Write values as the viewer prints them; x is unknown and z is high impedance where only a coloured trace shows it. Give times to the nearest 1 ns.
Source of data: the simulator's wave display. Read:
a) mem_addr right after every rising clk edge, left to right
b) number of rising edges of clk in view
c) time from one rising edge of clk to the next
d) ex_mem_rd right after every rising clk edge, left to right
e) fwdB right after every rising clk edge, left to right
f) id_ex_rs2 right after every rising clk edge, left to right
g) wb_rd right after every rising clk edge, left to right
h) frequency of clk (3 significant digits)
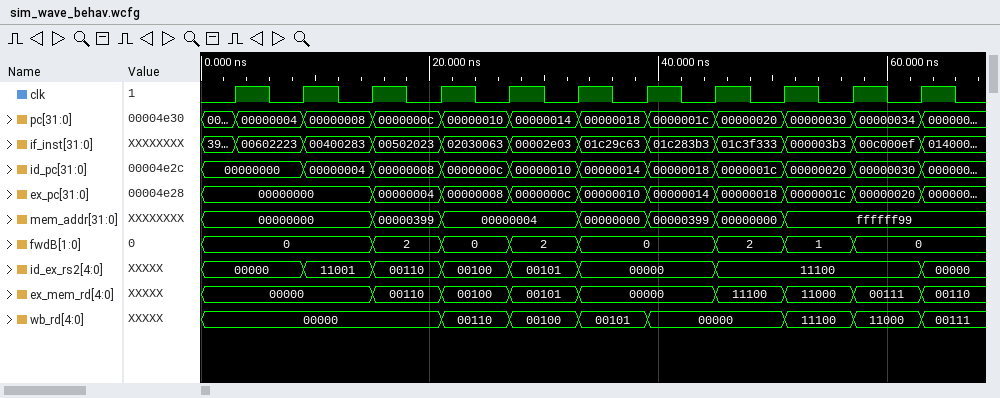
00000000, 00000000, 00000399, 00000004, 00000004, 00000000, 00000399, 00000000, ffffff99, ffffff99, ffffff99
11
6 ns
00000, 00000, 00110, 00100, 00101, 00000, 00000, 11100, 11000, 00111, 00110
0, 0, 2, 0, 2, 0, 0, 2, 1, 0, 0
00000, 11001, 00110, 00100, 00101, 00000, 00000, 11100, 11100, 11100, 00000
00000, 00000, 00000, 00110, 00100, 00101, 00000, 00000, 11100, 11000, 00111
167 MHz
